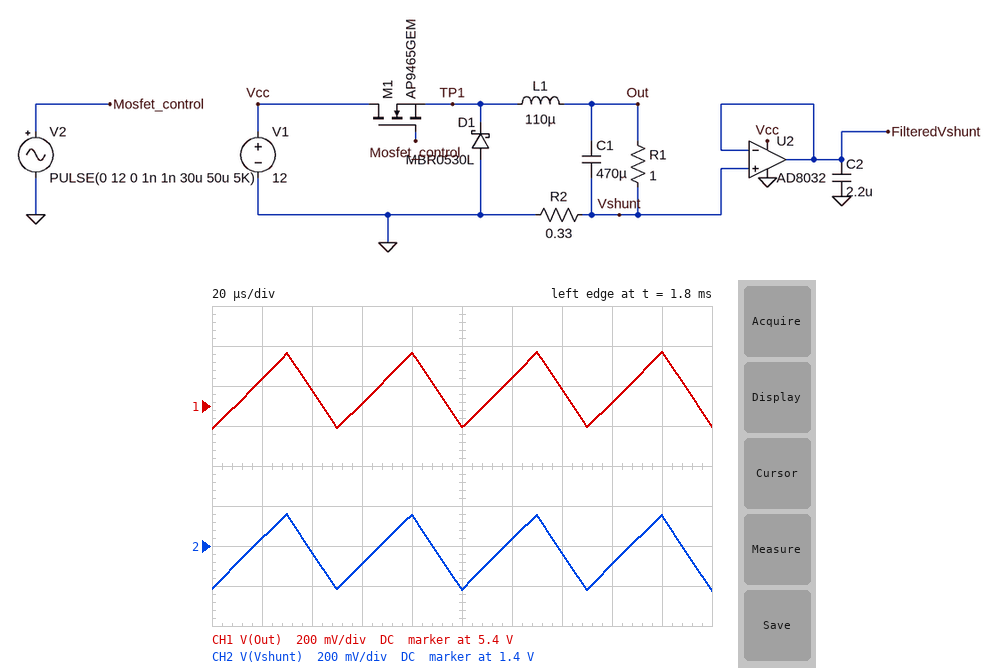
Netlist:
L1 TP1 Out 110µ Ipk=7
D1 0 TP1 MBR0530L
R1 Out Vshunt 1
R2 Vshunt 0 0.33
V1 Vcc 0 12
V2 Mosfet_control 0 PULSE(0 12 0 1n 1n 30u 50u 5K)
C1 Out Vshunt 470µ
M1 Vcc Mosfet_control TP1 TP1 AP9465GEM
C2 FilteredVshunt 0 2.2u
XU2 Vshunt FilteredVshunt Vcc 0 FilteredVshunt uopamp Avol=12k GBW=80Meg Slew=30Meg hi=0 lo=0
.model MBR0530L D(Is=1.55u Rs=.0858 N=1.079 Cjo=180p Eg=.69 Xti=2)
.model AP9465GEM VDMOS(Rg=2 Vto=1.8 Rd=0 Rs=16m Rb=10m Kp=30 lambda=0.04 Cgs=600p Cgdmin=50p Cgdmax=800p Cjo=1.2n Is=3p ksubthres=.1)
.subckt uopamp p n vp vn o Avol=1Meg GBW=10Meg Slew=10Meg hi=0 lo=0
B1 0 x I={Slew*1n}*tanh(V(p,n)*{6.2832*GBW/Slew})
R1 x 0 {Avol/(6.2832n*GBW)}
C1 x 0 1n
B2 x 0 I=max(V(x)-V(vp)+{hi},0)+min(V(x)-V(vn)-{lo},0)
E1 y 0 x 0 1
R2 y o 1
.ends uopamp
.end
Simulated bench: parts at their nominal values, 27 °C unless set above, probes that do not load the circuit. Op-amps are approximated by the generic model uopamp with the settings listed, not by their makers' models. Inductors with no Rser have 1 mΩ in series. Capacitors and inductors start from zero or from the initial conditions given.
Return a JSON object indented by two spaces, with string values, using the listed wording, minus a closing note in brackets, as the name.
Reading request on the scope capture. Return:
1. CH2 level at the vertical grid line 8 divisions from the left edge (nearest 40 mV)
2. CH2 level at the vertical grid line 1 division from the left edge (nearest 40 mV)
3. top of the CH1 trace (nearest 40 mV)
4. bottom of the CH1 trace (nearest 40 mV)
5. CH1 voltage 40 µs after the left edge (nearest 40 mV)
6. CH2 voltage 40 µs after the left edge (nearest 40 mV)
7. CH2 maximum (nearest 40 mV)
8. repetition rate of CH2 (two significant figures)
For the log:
{
  "CH2 level at the vertical grid line 8 divisions from the left edge": "1.32 V",
  "CH2 level at the vertical grid line 1 division from the left edge": "1.44 V",
  "top of the CH1 trace": "5.68 V",
  "bottom of the CH1 trace": "5.28 V",
  "CH1 voltage 40 µs after the left edge": "5.48 V",
  "CH2 voltage 40 µs after the left edge": "1.36 V",
  "CH2 maximum": "1.56 V",
  "repetition rate of CH2": "20 kHz"
}
